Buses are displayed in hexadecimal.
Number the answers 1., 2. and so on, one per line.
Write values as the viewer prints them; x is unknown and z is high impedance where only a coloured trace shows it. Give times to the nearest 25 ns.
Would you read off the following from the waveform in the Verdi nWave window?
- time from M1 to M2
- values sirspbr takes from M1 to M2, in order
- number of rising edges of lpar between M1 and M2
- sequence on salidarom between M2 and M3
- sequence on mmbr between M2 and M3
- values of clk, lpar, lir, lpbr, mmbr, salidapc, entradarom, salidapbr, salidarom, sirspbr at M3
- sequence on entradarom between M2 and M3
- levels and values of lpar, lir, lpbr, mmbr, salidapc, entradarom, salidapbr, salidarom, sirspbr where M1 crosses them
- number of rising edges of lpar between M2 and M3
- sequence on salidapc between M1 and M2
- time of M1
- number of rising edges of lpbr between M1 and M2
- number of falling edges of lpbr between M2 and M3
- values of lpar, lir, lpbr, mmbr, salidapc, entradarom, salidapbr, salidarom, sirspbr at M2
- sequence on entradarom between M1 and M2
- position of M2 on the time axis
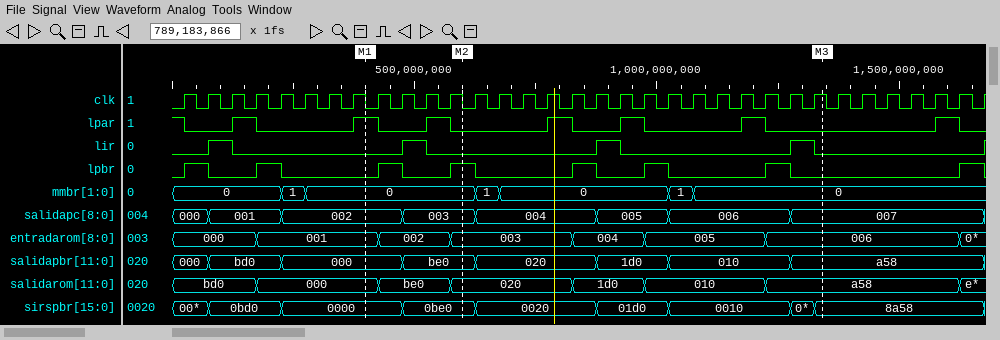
1. 200 ns
2. 0000, 0be0
3. 1
4. 020, 1d0, 010, a58
5. 0, 1, 0, 1, 0
6. clk=1, lpar=0, lir=0, lpbr=0, mmbr=0, salidapc=007, entradarom=006, salidapbr=a58, salidarom=a58, sirspbr=8a58
7. 003, 004, 005, 006
8. lpar=1, lir=0, lpbr=0, mmbr=0, salidapc=002, entradarom=001, salidapbr=000, salidarom=000, sirspbr=0000
9. 3
10. 002, 003
11. 400 ns
12. 2
13. 4
14. lpar=0, lir=0, lpbr=1, mmbr=0, salidapc=003, entradarom=003, salidapbr=be0, salidarom=020, sirspbr=0be0
15. 001, 002, 003
16. 600 ns
